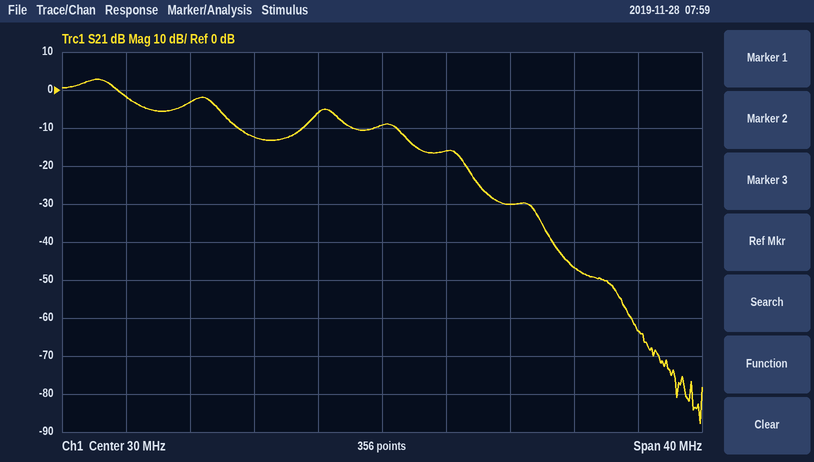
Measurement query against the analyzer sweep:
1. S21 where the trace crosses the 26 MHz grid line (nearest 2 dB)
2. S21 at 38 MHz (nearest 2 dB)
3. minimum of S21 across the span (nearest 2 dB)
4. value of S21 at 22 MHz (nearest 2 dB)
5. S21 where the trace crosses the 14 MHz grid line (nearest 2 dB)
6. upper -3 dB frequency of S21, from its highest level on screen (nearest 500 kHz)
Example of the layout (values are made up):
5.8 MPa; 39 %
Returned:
-6 dB; -30 dB; -88 dB; -12 dB; -2 dB; 13.5 MHz
